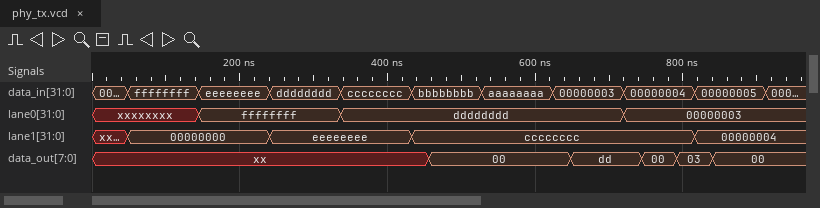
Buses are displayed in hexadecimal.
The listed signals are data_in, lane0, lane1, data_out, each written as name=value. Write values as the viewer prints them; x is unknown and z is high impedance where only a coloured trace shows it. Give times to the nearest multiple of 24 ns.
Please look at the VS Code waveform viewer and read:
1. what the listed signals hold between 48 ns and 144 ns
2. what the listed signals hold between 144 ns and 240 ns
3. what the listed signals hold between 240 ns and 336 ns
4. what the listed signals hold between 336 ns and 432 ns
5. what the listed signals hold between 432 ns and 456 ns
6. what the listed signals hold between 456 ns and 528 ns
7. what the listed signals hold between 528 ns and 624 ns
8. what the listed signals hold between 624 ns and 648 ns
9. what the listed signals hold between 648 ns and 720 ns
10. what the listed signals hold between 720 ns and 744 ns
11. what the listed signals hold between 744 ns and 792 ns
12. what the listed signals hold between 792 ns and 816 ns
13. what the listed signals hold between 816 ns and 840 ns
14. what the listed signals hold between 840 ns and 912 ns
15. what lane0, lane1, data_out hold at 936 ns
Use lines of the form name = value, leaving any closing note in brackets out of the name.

what the listed signals hold between 48 ns and 144 ns = data_in=ffffffff, lane0=xxxxxxxx, lane1=00000000, data_out=xx
what the listed signals hold between 144 ns and 240 ns = data_in=eeeeeeee, lane0=ffffffff, lane1=00000000, data_out=xx
what the listed signals hold between 240 ns and 336 ns = data_in=dddddddd, lane0=ffffffff, lane1=eeeeeeee, data_out=xx
what the listed signals hold between 336 ns and 432 ns = data_in=cccccccc, lane0=dddddddd, lane1=eeeeeeee, data_out=xx
what the listed signals hold between 432 ns and 456 ns = data_in=bbbbbbbb, lane0=dddddddd, lane1=cccccccc, data_out=xx
what the listed signals hold between 456 ns and 528 ns = data_in=bbbbbbbb, lane0=dddddddd, lane1=cccccccc, data_out=00
what the listed signals hold between 528 ns and 624 ns = data_in=aaaaaaaa, lane0=dddddddd, lane1=cccccccc, data_out=00
what the listed signals hold between 624 ns and 648 ns = data_in=00000003, lane0=dddddddd, lane1=cccccccc, data_out=00
what the listed signals hold between 648 ns and 720 ns = data_in=00000003, lane0=dddddddd, lane1=cccccccc, data_out=dd
what the listed signals hold between 720 ns and 744 ns = data_in=00000004, lane0=00000003, lane1=cccccccc, data_out=dd
what the listed signals hold between 744 ns and 792 ns = data_in=00000004, lane0=00000003, lane1=cccccccc, data_out=00
what the listed signals hold between 792 ns and 816 ns = data_in=00000004, lane0=00000003, lane1=cccccccc, data_out=03
what the listed signals hold between 816 ns and 840 ns = data_in=00000005, lane0=00000003, lane1=00000004, data_out=03
what the listed signals hold between 840 ns and 912 ns = data_in=00000005, lane0=00000003, lane1=00000004, data_out=00
what lane0, lane1, data_out hold at 936 ns = lane0=00000003, lane1=00000004, data_out=00
